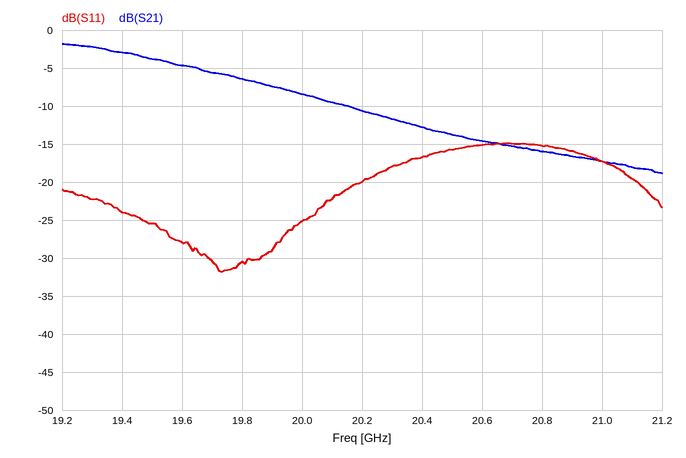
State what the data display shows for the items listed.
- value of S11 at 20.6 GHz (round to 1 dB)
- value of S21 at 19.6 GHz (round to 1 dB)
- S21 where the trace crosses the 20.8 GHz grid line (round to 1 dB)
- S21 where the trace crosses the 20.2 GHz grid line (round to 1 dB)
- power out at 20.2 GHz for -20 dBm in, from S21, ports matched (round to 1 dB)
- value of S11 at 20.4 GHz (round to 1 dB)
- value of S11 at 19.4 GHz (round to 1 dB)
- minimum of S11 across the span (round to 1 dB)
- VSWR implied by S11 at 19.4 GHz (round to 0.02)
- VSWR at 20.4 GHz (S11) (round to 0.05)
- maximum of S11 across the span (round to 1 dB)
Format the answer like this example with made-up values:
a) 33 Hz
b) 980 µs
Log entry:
a) -15 dB
b) -5 dB
c) -16 dB
d) -11 dB
e) -31 dBm
f) -17 dB
g) -24 dB
h) -32 dB
i) 1.14
j) 1.35
k) -15 dB
